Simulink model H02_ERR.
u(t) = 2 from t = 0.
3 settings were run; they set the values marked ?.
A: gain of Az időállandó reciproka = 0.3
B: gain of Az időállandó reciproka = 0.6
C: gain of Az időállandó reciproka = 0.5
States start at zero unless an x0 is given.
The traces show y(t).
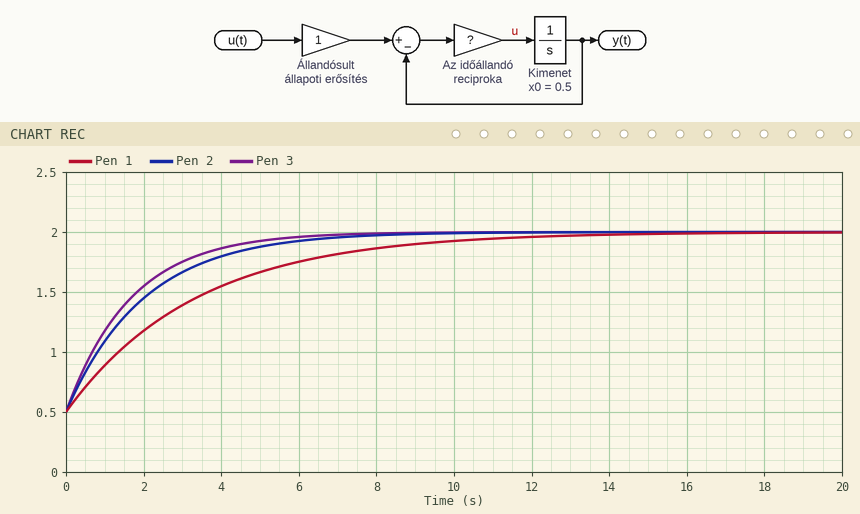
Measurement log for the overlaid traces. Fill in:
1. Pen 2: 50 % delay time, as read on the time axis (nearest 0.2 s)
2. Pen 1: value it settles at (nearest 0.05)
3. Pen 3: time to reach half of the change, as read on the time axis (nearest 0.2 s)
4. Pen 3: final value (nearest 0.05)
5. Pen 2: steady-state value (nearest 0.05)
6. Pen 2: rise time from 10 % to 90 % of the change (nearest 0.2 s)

1.4 s
2.00
1.2 s
2.00
2.00
4.4 s
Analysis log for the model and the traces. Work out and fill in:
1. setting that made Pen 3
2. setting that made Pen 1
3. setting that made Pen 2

B
A
C
